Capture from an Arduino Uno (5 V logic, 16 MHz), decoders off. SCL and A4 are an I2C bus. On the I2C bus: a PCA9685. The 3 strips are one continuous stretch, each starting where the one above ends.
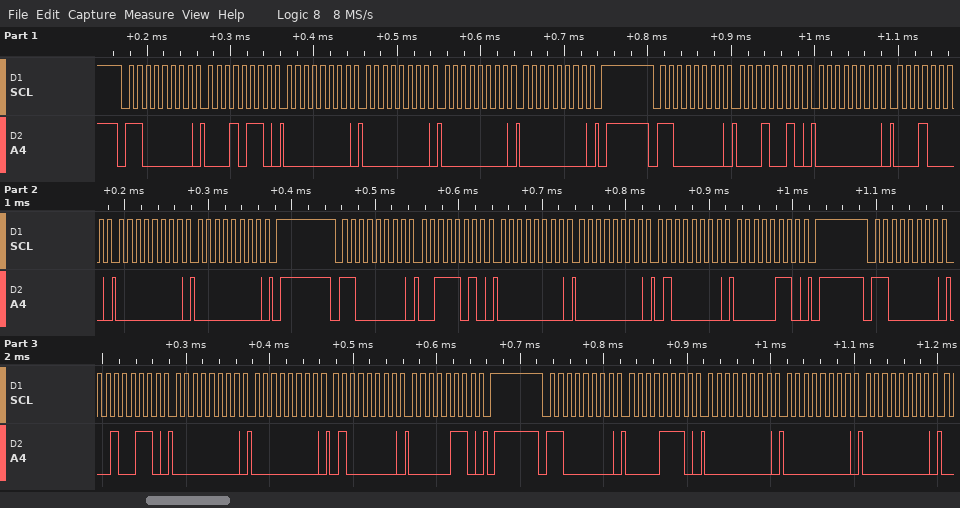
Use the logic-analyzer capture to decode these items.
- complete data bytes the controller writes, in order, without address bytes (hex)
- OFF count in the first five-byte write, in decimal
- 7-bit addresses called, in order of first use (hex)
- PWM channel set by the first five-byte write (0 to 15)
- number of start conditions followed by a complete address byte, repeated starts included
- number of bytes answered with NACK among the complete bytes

16 00 00 00 00 12 00 10 00 00 3A 00 00 40 06 26 00 00 40 06 0E 00 00 00
0
0x60
4
5
0
